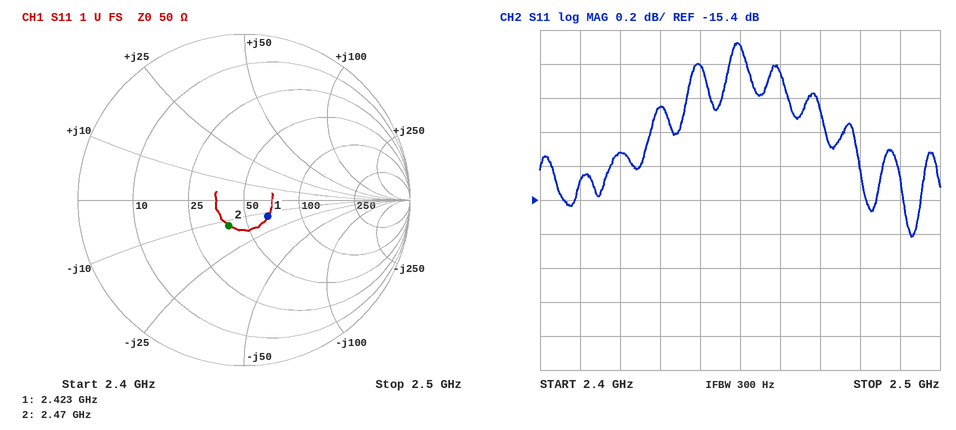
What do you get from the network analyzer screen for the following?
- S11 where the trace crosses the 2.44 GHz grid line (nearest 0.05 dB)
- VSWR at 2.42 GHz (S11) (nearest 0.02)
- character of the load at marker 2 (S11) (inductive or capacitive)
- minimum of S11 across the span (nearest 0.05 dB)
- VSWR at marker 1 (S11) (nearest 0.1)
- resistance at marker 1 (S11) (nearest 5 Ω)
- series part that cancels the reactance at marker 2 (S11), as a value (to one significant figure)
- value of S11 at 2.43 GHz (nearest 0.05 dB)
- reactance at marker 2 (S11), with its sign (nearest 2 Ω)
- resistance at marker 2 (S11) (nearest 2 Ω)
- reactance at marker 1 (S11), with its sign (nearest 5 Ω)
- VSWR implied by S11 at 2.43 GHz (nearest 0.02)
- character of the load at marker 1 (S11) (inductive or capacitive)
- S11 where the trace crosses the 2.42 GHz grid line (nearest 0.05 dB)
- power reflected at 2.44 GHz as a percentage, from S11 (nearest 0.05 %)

-14.60 dB
1.42
capacitive
-15.60 dB
1.4
65 Ω
800 pH
-14.85 dB
-12 Ω
40 Ω
-15 Ω
1.44
capacitive
-15.10 dB
3.45 %
